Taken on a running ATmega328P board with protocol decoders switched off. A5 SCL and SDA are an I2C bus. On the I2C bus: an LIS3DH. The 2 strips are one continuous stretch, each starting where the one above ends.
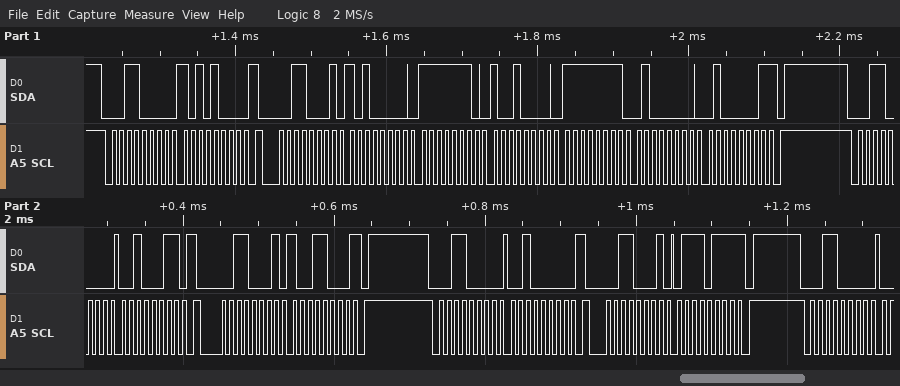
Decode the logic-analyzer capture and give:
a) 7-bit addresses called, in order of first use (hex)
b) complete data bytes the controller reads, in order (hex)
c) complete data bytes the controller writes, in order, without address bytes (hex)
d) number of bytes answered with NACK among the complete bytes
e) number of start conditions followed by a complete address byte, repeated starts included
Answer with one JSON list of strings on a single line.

["0x18", "A0 FE 90 FF 40 41 98 77", "A8 23 20", "3", "7"]
